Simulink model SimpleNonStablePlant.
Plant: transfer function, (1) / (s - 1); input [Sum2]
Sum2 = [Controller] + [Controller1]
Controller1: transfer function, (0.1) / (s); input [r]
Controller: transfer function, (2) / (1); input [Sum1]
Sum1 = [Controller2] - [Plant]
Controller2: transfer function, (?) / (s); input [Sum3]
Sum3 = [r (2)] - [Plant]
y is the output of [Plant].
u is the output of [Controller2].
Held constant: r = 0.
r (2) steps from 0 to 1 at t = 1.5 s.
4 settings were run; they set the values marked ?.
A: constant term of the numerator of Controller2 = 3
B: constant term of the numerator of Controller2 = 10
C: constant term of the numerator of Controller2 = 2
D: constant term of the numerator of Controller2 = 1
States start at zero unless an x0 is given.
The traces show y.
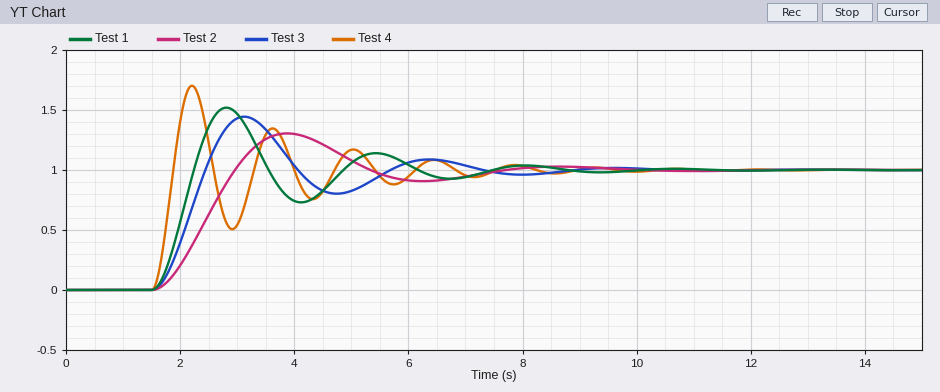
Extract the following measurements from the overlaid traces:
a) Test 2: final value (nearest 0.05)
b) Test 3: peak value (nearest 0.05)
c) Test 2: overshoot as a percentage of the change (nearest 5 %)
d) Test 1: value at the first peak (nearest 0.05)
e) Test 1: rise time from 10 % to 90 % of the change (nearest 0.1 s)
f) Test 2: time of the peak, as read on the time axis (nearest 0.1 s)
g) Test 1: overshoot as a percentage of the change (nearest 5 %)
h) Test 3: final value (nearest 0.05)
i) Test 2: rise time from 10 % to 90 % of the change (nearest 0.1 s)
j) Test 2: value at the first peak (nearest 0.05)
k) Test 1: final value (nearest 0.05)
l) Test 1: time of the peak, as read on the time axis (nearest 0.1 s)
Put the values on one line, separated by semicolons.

1.00; 1.45; 30 %; 1.50; 0.5 s; 3.9 s; 50 %; 1.00; 1.0 s; 1.30; 1.00; 2.8 s
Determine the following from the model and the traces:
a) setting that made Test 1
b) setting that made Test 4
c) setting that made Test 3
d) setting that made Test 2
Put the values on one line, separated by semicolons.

A; B; C; D
